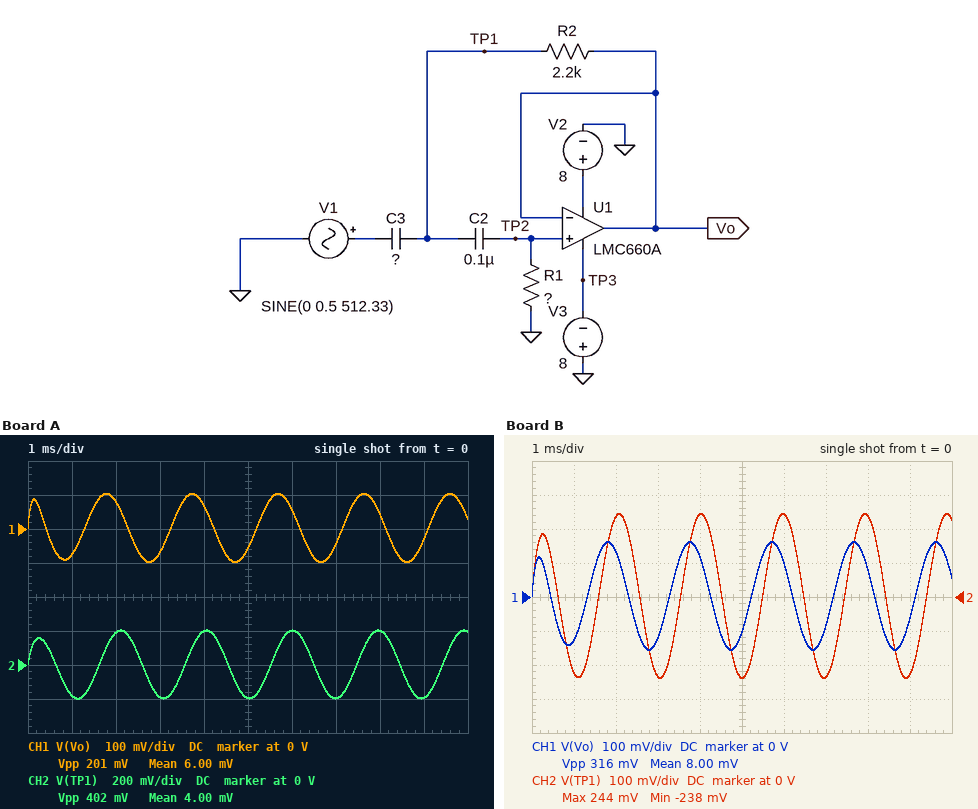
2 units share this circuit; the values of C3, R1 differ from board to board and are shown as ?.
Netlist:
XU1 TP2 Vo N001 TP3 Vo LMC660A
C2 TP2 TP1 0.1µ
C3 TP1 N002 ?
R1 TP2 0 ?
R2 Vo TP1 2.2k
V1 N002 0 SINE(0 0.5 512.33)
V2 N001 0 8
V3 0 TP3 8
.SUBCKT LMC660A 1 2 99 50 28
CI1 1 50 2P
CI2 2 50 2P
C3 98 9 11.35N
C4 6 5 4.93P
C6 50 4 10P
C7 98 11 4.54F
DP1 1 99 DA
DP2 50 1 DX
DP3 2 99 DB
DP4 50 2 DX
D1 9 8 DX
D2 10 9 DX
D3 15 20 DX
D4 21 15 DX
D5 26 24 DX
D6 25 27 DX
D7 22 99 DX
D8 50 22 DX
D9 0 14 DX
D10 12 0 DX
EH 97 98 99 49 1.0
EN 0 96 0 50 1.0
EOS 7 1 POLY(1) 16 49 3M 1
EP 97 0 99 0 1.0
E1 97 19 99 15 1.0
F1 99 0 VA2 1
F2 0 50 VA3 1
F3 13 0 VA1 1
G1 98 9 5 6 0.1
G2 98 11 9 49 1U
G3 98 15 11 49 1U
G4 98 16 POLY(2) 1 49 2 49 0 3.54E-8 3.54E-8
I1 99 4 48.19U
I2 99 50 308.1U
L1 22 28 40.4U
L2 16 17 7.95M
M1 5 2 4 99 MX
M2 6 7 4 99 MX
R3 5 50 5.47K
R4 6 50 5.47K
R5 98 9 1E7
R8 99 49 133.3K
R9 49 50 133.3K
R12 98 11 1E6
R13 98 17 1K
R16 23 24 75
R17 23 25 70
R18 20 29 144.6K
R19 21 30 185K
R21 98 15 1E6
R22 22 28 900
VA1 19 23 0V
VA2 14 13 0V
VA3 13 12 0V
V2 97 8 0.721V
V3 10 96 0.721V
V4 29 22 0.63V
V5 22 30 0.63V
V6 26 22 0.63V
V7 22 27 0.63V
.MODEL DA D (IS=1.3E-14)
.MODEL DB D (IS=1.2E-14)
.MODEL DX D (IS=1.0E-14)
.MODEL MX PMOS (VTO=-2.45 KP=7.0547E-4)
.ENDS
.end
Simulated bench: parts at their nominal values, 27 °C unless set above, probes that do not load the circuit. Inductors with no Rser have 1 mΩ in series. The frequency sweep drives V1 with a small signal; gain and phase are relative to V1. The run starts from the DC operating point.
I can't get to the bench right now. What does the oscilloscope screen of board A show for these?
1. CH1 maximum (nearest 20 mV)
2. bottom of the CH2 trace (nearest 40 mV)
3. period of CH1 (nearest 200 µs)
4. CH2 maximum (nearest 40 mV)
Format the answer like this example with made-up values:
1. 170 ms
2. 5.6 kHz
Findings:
1. 100 mV
2. -200 mV
3. 2.0 ms
4. 200 mV
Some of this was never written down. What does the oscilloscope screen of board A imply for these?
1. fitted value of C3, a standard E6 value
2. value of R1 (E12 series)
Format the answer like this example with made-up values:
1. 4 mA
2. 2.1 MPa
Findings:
1. 68 nF
2. 1.8 kΩ
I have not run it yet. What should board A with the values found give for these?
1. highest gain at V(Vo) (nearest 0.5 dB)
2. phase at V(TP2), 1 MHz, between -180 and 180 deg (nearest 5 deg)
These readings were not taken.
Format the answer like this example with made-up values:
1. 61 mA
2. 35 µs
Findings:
1. 0 dB
2. 0 deg
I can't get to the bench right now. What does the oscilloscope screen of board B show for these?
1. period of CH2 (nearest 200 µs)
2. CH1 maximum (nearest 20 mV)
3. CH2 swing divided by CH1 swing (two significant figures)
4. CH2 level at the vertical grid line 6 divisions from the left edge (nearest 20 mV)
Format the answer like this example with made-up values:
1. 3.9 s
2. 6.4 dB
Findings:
1. 2.0 ms
2. 160 mV
3. 1.5
4. 240 mV
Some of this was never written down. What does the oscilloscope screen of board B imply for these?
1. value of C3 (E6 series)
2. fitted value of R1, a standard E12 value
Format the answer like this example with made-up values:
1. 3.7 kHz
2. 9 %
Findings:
1. 68 nF
2. 2.7 kΩ
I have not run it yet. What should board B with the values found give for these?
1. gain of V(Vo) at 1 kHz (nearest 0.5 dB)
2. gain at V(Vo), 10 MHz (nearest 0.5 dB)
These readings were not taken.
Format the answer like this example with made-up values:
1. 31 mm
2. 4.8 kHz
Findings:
1. -3.5 dB
2. -11.0 dB
